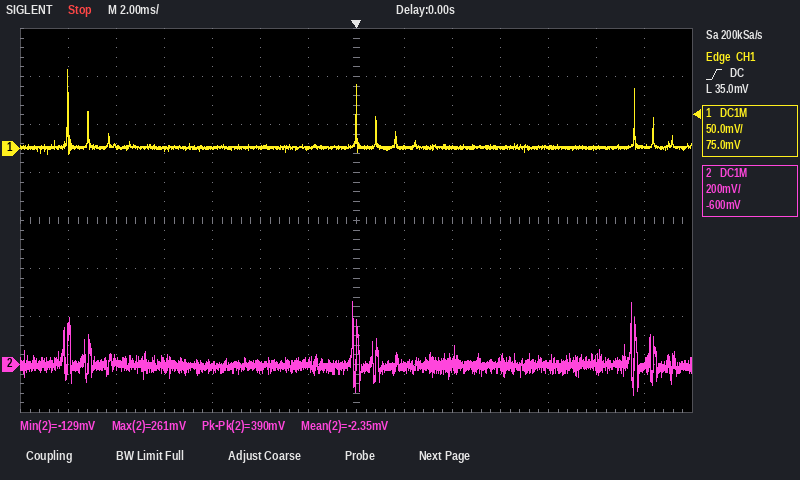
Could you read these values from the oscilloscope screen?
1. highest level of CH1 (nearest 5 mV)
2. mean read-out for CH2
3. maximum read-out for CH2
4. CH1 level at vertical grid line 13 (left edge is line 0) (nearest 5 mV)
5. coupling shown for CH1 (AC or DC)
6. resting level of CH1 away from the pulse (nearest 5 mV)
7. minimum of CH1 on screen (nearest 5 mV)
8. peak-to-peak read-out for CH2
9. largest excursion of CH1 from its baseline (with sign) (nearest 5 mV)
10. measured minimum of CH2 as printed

80 mV
-2.35 mV
261 mV
0 mV
DC
0 mV
-5 mV
390 mV
+80 mV
-129 mV
